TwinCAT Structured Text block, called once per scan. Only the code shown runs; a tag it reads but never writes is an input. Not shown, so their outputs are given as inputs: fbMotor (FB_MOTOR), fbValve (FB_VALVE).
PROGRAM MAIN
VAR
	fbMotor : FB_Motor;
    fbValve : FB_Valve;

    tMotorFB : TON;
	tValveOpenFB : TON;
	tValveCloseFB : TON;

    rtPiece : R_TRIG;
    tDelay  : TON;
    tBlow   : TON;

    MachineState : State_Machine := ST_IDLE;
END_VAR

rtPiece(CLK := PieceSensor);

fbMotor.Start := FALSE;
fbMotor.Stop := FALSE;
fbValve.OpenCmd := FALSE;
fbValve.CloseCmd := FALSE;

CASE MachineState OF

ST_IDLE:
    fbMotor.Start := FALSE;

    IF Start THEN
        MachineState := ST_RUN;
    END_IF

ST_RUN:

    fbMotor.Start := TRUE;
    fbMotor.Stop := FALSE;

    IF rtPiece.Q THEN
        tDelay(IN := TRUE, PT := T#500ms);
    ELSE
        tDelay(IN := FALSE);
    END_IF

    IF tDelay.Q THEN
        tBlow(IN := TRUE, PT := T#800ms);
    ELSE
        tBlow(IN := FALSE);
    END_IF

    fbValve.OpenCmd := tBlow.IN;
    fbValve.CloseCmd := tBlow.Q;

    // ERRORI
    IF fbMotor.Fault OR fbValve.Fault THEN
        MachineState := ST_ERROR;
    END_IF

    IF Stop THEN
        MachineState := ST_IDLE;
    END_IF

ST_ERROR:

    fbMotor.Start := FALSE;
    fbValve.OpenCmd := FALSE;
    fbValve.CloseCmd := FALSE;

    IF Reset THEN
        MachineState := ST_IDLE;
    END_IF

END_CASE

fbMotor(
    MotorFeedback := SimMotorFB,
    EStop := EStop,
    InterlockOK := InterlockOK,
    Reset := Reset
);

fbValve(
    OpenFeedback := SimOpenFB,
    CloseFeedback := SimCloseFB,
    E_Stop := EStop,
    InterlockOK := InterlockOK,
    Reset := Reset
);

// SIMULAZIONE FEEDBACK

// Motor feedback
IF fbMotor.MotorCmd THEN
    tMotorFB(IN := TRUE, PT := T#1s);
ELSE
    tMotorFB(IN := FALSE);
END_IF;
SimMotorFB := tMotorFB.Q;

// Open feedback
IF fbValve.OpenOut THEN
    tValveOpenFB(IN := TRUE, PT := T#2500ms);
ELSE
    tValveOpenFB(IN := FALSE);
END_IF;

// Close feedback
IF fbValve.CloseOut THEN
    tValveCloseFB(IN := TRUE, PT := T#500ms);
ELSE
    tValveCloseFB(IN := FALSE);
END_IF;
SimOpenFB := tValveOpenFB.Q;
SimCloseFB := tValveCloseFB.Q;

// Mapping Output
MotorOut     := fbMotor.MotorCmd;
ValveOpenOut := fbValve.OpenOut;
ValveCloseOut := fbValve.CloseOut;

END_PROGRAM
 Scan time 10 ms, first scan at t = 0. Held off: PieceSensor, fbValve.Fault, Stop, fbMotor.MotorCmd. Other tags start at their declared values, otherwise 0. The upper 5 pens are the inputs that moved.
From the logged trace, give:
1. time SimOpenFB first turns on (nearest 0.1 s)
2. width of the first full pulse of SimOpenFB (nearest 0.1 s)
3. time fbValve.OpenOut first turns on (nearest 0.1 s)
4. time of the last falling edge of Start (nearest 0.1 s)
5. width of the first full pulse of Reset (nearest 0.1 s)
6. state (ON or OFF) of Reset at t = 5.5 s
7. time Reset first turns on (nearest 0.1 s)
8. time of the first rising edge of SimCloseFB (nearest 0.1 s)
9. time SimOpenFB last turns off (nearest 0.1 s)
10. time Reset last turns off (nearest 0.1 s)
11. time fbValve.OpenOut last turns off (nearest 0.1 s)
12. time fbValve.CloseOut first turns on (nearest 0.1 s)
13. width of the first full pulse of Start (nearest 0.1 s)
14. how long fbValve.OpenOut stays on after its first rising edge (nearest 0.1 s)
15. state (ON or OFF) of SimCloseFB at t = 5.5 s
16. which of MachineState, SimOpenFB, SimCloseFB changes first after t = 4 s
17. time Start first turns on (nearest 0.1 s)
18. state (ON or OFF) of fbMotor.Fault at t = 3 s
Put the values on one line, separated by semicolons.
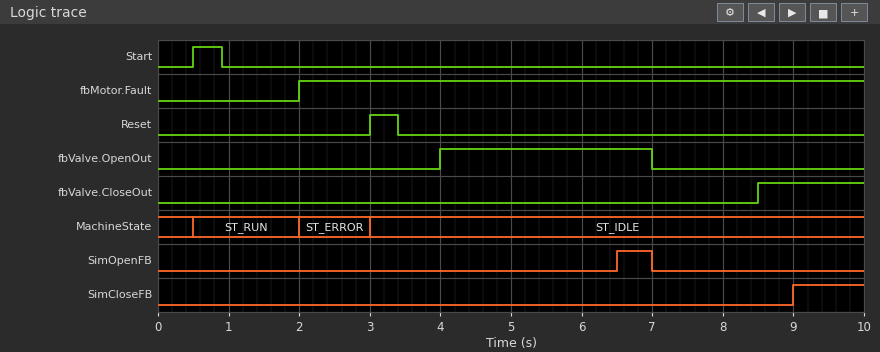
6.5 s; 0.5 s; 4.0 s; 0.9 s; 0.4 s; OFF; 3.0 s; 9.0 s; 7.0 s; 3.4 s; 7.0 s; 8.5 s; 0.4 s; 3.0 s; OFF; SimOpenFB; 0.5 s; ON
